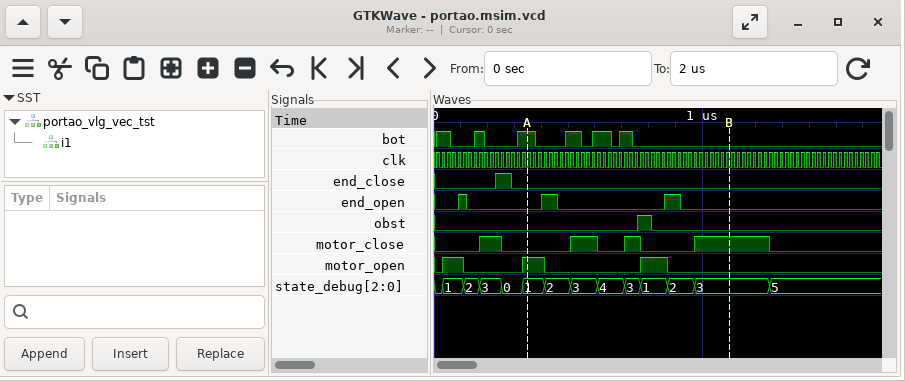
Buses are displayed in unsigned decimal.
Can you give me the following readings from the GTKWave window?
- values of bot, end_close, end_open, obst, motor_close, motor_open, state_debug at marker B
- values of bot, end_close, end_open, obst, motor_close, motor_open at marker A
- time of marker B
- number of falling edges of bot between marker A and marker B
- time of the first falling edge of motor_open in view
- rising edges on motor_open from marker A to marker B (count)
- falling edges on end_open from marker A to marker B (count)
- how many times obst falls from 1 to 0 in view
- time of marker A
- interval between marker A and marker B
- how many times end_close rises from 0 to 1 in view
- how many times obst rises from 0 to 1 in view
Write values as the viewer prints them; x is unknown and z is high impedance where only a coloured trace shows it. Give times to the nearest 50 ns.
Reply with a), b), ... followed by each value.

a) bot=0, end_close=0, end_open=0, obst=0, motor_close=1, motor_open=0, state_debug=3
b) bot=1, end_close=0, end_open=0, obst=0, motor_close=0, motor_open=1
c) 1100 ns
d) 4
e) 100 ns
f) 1
g) 2
h) 1
i) 350 ns
j) 750 ns
k) 1
l) 1
